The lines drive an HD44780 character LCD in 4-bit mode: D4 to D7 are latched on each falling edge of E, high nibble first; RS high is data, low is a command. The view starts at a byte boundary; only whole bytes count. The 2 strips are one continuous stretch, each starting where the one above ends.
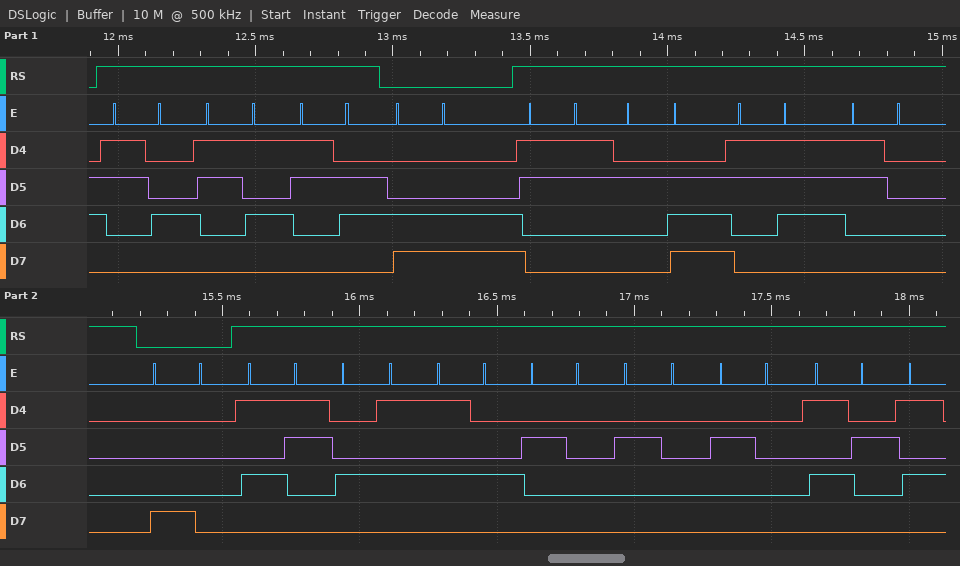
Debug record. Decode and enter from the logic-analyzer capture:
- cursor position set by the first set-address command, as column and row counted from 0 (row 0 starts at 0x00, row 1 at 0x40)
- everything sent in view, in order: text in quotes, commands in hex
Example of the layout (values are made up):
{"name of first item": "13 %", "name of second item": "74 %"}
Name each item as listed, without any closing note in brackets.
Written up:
{"cursor position set by the first set-address command, as column and row counted from 0": "column 12, row 1", "everything sent in view, in order: text in quotes, commands in hex": "\"456\" 0xCC \"3.70\" 0x80 \"SET   R\""}
